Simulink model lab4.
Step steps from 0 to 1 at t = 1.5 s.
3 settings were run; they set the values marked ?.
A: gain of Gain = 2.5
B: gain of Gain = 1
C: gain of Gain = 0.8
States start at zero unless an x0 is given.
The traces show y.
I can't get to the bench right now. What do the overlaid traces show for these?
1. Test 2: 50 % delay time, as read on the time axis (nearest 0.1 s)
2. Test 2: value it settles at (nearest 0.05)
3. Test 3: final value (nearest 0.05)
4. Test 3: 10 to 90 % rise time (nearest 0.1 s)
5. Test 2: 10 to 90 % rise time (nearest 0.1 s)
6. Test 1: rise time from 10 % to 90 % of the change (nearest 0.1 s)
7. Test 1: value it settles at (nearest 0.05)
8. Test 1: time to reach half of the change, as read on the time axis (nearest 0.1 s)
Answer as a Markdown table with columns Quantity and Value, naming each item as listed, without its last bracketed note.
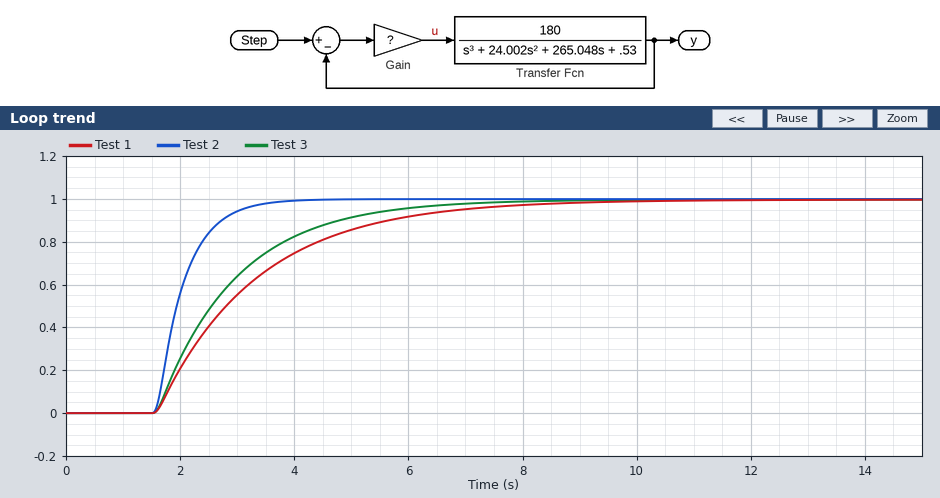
| Quantity | Value |
|---|---|
| Test 2: 50 % delay time, as read on the time axis | 1.9 s |
| Test 2: value it settles at | 1.00 |
| Test 3: final value | 1.00 |
| Test 3: 10 to 90 % rise time | 3.0 s |
| Test 2: 10 to 90 % rise time | 1.1 s |
| Test 1: rise time from 10 % to 90 % of the change | 3.8 s |
| Test 1: value it settles at | 1.00 |
| Test 1: time to reach half of the change, as read on the time axis | 2.8 s |
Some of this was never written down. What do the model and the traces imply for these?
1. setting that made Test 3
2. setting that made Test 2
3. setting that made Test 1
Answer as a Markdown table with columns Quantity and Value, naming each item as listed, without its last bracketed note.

| Quantity | Value |
|---|---|
| setting that made Test 3 | B |
| setting that made Test 2 | A |
| setting that made Test 1 | C |
